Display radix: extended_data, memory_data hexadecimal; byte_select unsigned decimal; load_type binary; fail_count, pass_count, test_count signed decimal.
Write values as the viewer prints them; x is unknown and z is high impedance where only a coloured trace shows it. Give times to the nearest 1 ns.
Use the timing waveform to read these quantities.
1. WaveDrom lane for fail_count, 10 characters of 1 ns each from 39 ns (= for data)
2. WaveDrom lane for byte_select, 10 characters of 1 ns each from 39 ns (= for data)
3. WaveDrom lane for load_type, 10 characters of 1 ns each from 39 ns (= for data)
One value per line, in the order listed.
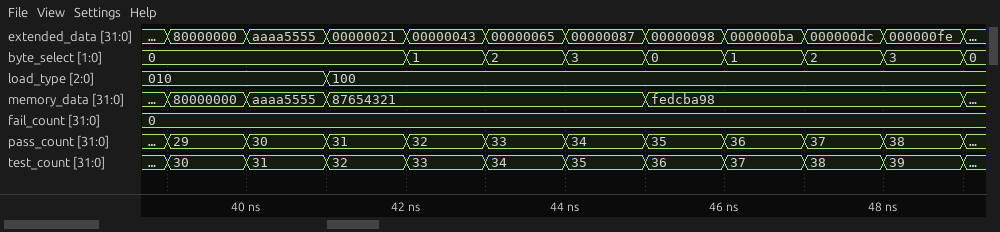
{name: 'fail_count', wave: '=.........', data: '0'}
{name: 'byte_select', wave: '=..=======', data: '0 1 2 3 0 1 2 3'}
{name: 'load_type', wave: '=.=.......', data: '010 100'}
